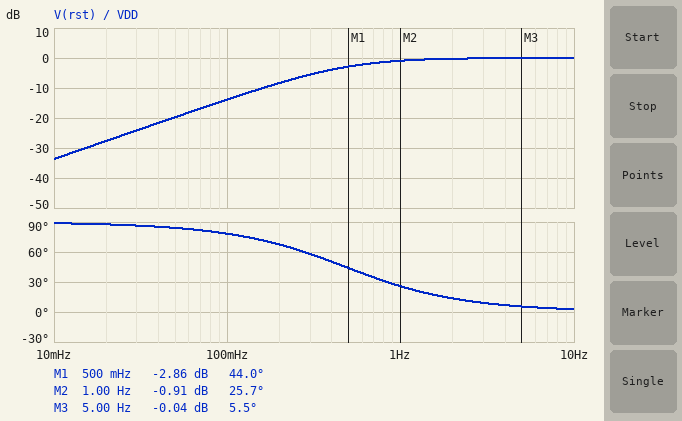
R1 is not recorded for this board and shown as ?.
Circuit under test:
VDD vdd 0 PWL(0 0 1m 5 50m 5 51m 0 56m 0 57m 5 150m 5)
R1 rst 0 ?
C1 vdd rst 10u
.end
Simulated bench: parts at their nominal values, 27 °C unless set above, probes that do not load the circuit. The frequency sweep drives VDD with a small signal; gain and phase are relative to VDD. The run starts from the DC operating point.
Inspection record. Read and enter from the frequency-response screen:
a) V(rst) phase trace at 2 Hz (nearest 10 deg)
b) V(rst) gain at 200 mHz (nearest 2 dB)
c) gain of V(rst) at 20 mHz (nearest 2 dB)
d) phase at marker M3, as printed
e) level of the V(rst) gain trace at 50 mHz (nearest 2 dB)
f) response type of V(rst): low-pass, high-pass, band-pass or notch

10 deg
-8 dB
-28 dB
5.5 deg
-20 dB
high-pass
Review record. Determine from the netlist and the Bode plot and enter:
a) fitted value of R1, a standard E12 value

33 kΩ
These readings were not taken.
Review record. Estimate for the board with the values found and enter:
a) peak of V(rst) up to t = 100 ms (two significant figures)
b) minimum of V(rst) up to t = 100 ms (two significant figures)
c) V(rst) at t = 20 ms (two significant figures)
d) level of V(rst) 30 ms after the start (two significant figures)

5.0 V
-700 mV
4.7 V
4.6 V
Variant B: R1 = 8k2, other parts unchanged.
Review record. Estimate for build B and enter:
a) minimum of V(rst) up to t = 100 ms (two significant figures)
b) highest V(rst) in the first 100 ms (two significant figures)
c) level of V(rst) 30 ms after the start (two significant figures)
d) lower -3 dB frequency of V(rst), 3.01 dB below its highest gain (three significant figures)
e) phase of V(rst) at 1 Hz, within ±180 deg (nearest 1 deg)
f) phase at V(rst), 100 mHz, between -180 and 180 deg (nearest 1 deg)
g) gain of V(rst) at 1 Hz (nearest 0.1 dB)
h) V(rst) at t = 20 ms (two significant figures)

-2.3 V
5.0 V
3.5 V
1.94 Hz
63 deg
87 deg
-6.8 dB
3.9 V
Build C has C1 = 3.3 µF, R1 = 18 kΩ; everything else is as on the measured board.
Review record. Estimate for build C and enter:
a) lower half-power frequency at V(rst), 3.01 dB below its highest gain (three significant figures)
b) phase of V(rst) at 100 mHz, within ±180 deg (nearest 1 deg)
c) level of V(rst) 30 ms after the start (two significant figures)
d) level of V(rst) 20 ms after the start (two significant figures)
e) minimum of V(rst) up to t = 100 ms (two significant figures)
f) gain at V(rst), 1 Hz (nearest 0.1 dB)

2.68 Hz
88 deg
3.0 V
3.6 V
-2.8 V
-9.1 dB
